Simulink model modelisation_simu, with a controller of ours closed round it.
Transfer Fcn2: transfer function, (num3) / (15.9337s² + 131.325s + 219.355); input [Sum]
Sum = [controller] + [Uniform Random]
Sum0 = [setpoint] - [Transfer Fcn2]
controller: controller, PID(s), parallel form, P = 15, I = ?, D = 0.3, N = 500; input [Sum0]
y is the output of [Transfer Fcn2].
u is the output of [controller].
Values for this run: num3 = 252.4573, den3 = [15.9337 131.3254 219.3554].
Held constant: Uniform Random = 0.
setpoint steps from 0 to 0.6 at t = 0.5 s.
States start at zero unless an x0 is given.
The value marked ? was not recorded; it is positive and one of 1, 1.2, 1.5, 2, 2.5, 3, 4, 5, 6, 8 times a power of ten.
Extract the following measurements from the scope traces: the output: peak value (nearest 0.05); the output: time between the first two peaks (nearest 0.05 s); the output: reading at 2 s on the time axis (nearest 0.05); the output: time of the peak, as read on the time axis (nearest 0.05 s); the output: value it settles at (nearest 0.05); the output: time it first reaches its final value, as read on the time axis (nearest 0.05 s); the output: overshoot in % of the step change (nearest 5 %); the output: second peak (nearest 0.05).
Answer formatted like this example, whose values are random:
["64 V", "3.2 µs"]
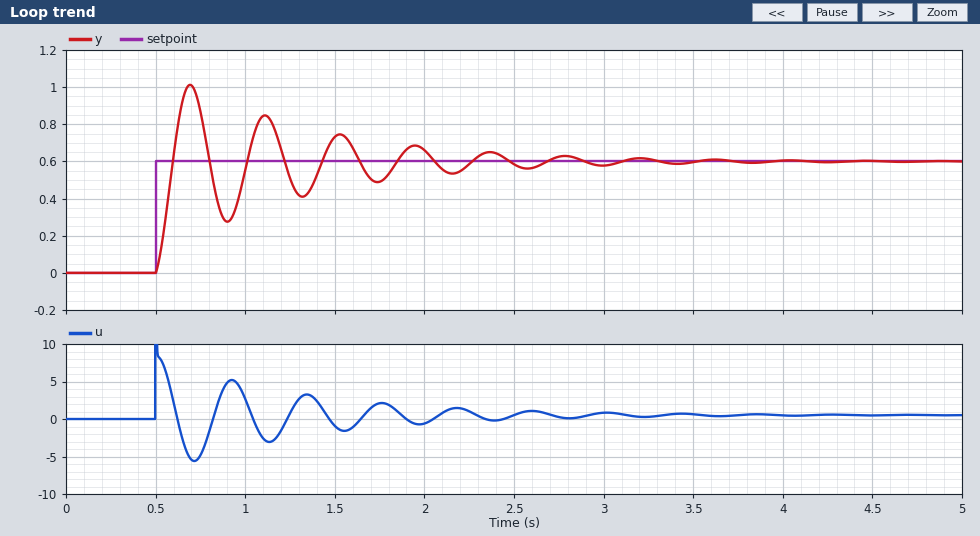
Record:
["1.00", "0.40 s", "0.65", "0.70 s", "0.60", "0.60 s", "70 %", "0.85"]
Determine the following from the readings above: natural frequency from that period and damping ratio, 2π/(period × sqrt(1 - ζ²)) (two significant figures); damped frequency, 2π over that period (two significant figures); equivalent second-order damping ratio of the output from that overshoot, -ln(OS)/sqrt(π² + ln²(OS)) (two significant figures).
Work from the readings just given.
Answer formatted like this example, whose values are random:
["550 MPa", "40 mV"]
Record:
["16 rad/s", "16 rad/s", "0.11"]
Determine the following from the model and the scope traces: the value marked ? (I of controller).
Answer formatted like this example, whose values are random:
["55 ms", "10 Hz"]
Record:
["150"]
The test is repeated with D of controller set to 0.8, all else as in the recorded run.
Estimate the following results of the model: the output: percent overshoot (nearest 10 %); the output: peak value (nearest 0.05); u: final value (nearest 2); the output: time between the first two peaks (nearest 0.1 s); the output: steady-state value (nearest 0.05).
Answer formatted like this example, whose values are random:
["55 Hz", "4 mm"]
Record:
["40 %", "0.85", "0", "0.5 s", "0.60"]
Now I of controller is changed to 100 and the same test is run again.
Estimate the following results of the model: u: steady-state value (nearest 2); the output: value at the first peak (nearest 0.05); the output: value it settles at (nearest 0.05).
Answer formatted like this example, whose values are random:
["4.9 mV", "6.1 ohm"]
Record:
["0", "0.95", "0.60"]
